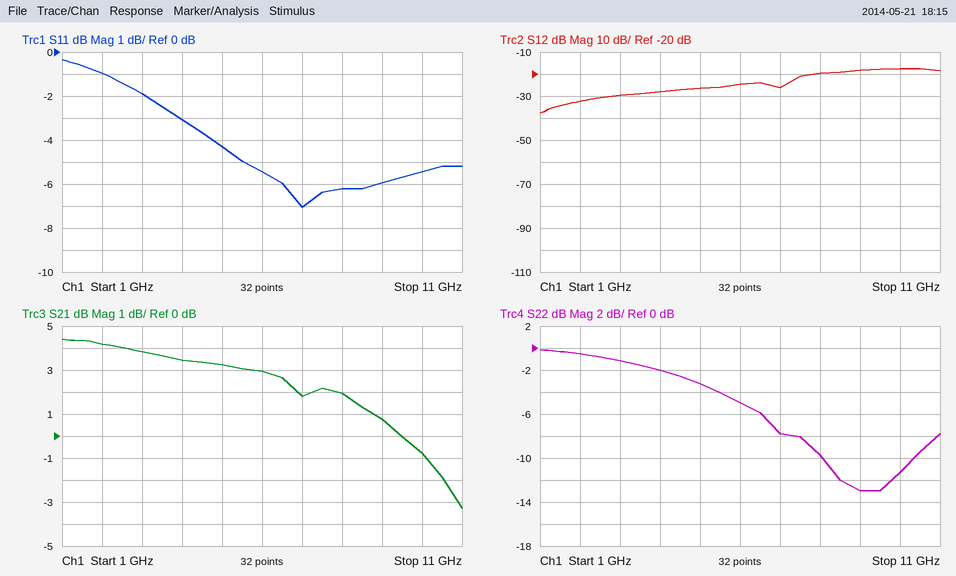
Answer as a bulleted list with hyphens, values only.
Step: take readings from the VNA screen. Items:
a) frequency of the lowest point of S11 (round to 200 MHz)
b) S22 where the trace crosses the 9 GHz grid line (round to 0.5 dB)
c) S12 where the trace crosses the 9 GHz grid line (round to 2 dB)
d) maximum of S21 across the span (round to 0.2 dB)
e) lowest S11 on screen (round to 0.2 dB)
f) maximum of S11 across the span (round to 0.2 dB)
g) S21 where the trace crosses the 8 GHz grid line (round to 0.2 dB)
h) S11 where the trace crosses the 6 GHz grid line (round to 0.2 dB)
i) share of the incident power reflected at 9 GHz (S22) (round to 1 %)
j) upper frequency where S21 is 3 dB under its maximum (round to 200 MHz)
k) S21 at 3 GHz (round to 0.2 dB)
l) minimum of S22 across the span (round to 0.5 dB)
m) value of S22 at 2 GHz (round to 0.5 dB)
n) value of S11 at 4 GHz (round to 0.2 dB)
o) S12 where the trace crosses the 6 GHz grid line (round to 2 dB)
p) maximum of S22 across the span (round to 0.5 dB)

- 7.0 GHz
- -13.0 dB
- -18 dB
- 4.4 dB
- -7.0 dB
- -0.4 dB
- 2.0 dB
- -5.4 dB
- 5 %
- 8.4 GHz
- 3.8 dB
- -13.0 dB
- -0.5 dB
- -3.0 dB
- -24 dB
- 0.0 dB
